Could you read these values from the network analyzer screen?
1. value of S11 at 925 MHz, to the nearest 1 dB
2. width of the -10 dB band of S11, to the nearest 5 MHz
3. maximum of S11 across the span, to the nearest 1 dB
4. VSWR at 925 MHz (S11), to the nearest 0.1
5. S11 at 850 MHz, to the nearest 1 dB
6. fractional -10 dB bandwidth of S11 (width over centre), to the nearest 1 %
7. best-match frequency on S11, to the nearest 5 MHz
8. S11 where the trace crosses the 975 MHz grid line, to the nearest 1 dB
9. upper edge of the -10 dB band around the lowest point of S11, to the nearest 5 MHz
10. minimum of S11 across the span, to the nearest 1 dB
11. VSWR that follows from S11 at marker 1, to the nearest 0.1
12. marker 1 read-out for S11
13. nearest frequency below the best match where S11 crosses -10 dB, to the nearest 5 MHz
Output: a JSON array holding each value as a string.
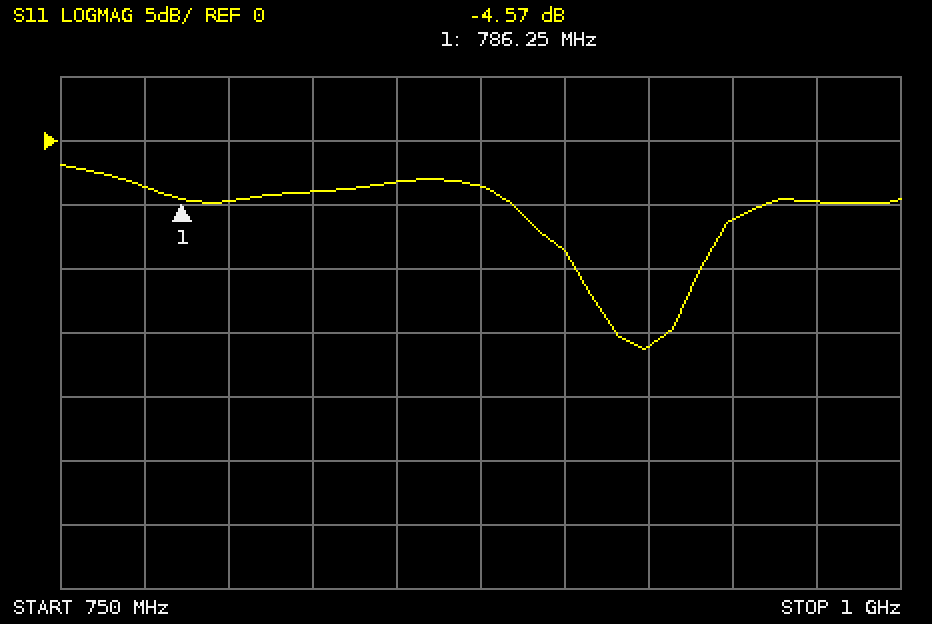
["-16 dB", "35 MHz", "-2 dB", "1.4", "-3 dB", "4 %", "925 MHz", "-5 dB", "940 MHz", "-16 dB", "3.9", "-4.57 dB", "905 MHz"]
